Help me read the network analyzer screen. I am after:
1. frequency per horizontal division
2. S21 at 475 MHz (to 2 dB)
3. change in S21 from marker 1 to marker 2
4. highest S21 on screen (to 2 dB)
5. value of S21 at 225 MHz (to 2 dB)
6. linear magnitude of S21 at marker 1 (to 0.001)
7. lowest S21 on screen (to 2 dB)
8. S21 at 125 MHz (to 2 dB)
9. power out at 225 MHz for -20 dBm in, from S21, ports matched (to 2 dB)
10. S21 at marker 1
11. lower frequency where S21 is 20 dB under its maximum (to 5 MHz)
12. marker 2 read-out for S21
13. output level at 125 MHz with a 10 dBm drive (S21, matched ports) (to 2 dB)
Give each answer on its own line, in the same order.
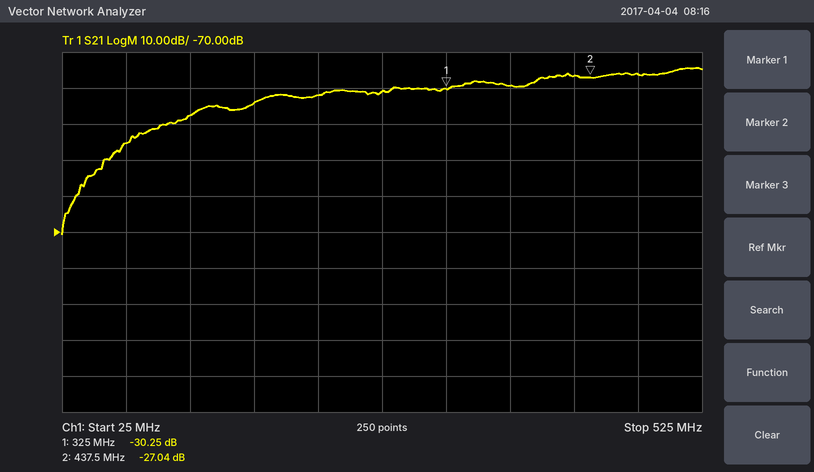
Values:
50 MHz
-26 dB
3.21 dB
-24 dB
-32 dB
0.031
-70 dB
-38 dB
-52 dBm
-30.25 dB
80 MHz
-27.04 dB
-28 dBm
